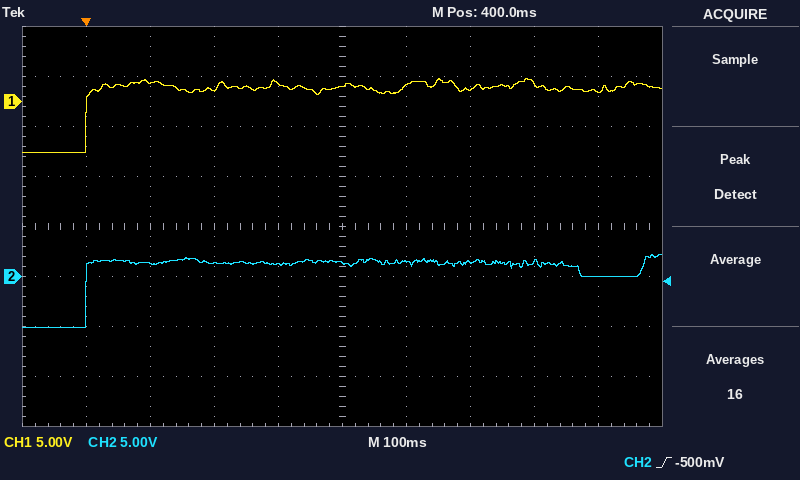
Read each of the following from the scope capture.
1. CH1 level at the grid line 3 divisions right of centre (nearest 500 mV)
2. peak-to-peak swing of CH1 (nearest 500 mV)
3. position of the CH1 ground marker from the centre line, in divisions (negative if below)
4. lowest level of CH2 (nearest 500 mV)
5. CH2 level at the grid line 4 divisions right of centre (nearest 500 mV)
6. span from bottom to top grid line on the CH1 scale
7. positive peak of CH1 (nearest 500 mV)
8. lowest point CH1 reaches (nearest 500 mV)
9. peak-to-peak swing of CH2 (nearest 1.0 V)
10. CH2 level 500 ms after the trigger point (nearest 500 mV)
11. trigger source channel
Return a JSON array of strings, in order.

["2.0 V", "7.5 V", "+2.5 div", "-5.0 V", "0.0 V", "40 V", "2.5 V", "-5.0 V", "7.0 V", "1.5 V", "CH2"]
